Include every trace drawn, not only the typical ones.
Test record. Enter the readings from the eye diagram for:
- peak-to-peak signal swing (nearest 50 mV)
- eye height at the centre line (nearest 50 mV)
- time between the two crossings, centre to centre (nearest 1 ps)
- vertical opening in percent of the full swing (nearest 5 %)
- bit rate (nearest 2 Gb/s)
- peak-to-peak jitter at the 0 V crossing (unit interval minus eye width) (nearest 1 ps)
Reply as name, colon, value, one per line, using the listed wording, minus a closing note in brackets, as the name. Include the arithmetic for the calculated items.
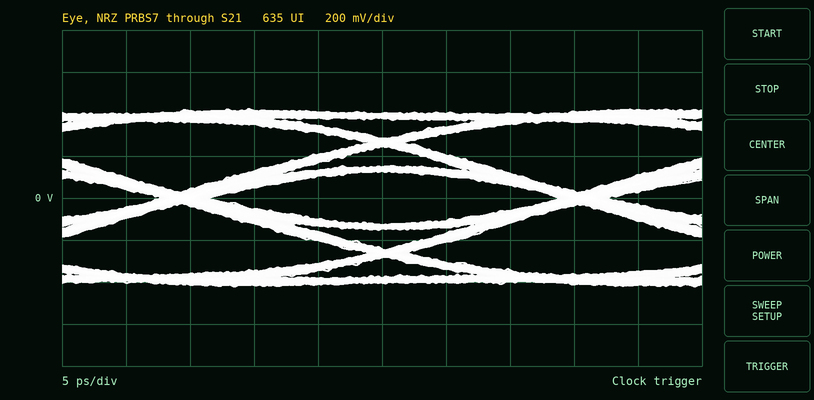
peak-to-peak signal swing: 850 mV
eye height at the centre line: 250 mV
time between the two crossings, centre to centre: 31 ps
vertical opening in percent of the full swing: 250 mV / 850 mV ≈ 29.4 %, so 30 % to the nearest 5 %
bit rate: 32 Gb/s
peak-to-peak jitter at the 0 V crossing (unit interval minus eye width): 4 ps
